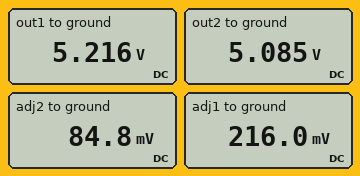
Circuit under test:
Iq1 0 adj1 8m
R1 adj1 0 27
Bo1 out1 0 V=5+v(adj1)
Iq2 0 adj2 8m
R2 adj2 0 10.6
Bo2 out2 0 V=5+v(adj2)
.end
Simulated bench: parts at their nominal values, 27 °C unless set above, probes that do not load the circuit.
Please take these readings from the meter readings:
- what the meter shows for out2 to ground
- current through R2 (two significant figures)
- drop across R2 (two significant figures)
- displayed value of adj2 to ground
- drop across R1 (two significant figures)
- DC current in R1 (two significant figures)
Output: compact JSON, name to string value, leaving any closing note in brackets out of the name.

{"what the meter shows for out2 to ground": "5.085 V", "current through R2": "8.0 mA", "drop across R2": "85 mV", "displayed value of adj2 to ground": "84.8 mV", "drop across R1": "220 mV", "DC current in R1": "8.0 mA"}
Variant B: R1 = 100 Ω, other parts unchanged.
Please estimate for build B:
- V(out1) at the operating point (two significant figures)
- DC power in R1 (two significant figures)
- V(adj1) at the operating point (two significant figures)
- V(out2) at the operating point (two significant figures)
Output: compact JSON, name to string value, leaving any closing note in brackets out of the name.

{"V(out1) at the operating point": "5.8 V", "DC power in R1": "6.4 mW", "V(adj1) at the operating point": "800 mV", "V(out2) at the operating point": "5.1 V"}
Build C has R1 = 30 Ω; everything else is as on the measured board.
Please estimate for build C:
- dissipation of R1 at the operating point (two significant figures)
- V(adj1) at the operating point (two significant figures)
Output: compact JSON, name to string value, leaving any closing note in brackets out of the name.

{"dissipation of R1 at the operating point": "1.9 mW", "V(adj1) at the operating point": "240 mV"}
